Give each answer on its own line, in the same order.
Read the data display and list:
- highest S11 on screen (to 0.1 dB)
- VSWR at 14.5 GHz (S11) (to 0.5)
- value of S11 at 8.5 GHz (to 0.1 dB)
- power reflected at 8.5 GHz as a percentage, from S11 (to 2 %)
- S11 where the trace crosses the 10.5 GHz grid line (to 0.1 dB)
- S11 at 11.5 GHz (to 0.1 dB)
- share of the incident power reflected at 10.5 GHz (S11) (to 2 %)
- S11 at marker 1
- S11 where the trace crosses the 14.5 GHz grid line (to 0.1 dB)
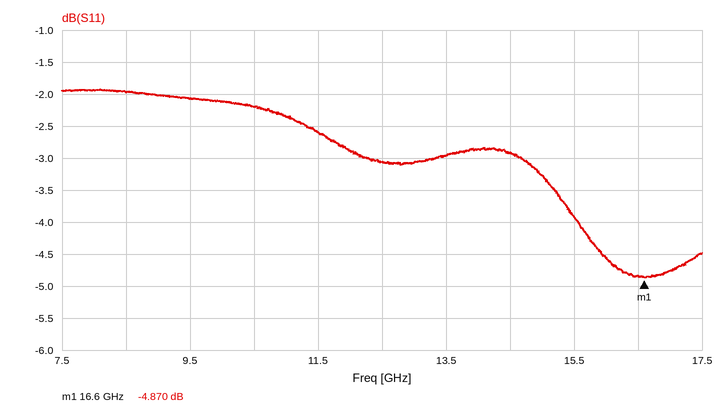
-1.9 dB
6.0
-2.0 dB
64 %
-2.2 dB
-2.6 dB
60 %
-4.870 dB
-2.9 dB
